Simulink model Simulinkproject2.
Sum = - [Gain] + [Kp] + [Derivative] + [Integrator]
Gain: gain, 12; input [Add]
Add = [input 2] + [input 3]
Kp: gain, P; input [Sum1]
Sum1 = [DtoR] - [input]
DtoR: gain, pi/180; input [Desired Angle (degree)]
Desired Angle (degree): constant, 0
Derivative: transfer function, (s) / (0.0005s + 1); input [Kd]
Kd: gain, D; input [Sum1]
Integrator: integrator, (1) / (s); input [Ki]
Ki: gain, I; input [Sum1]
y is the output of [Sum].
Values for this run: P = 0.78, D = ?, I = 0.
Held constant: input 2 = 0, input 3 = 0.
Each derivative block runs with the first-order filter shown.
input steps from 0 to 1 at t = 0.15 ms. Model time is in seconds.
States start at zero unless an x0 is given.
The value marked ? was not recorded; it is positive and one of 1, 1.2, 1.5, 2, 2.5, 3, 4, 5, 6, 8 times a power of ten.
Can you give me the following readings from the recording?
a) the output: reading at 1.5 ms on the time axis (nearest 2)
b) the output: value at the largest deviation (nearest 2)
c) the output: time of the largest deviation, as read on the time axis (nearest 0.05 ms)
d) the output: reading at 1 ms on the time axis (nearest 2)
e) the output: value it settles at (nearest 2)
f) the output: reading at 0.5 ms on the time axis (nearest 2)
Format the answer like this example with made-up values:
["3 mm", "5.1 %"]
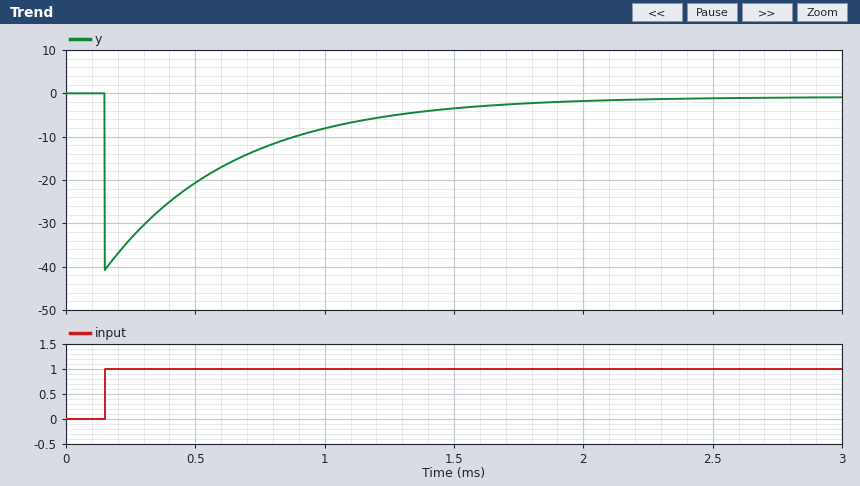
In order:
["-4", "-40", "0.15 ms", "-8", "0", "-20"]
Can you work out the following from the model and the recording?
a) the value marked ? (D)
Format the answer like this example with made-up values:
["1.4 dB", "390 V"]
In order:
["0.02"]
